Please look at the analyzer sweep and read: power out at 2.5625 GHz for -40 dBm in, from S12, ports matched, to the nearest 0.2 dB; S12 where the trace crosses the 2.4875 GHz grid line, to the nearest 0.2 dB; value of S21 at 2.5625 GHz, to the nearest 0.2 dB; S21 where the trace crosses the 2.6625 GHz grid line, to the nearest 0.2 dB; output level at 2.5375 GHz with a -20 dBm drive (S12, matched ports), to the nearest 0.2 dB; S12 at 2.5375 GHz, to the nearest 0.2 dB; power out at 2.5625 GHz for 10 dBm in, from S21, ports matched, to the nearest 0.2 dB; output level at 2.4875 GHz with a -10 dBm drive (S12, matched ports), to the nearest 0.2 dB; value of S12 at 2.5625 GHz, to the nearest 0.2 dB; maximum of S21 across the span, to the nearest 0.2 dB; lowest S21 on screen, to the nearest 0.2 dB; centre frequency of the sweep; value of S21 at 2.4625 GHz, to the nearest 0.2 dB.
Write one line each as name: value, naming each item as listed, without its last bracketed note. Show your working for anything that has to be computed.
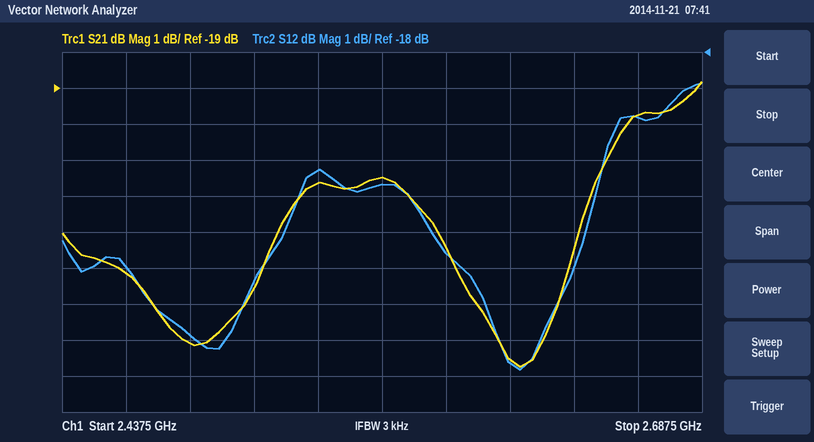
power out at 2.5625 GHz for -40 dBm in, from S12, ports matched, to the nearest 0.2 dB: -40 dBm + (-21.6 dB) = -61.6 dBm
S12 where the trace crosses the 2.4875 GHz grid line, to the nearest 0.2 dB: -25.8 dB
value of S21 at 2.5625 GHz, to the nearest 0.2 dB: -21.4 dB
S21 where the trace crosses the 2.6625 GHz grid line, to the nearest 0.2 dB: -19.8 dB
output level at 2.5375 GHz with a -20 dBm drive (S12, matched ports), to the nearest 0.2 dB: -20 dBm + (-21.2 dB) = -41.2 dBm
S12 at 2.5375 GHz, to the nearest 0.2 dB: -21.2 dB
power out at 2.5625 GHz for 10 dBm in, from S21, ports matched, to the nearest 0.2 dB: 10 dBm + (-21.4 dB) = -11.4 dBm
output level at 2.4875 GHz with a -10 dBm drive (S12, matched ports), to the nearest 0.2 dB: -10 dBm + (-25.8 dB) = -35.8 dBm
value of S12 at 2.5625 GHz, to the nearest 0.2 dB: -21.6 dB
maximum of S21 across the span, to the nearest 0.2 dB: -18.8 dB
lowest S21 on screen, to the nearest 0.2 dB: -26.8 dB
centre frequency of the sweep: 2.5625 GHz
value of S21 at 2.4625 GHz, to the nearest 0.2 dB: -24.2 dB
